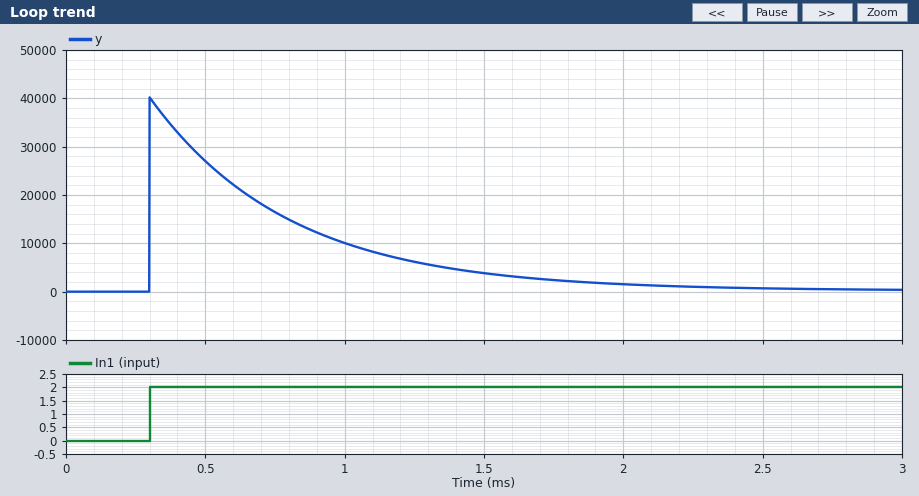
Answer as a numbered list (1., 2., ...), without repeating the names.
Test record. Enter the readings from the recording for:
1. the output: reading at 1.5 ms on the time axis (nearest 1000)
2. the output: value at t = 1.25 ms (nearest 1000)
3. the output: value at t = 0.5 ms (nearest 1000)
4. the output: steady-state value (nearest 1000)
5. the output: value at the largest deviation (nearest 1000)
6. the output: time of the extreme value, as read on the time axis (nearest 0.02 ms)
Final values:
1. 4000
2. 6000
3. 27000
4. 0
5. 40000
6. 0.30 ms
